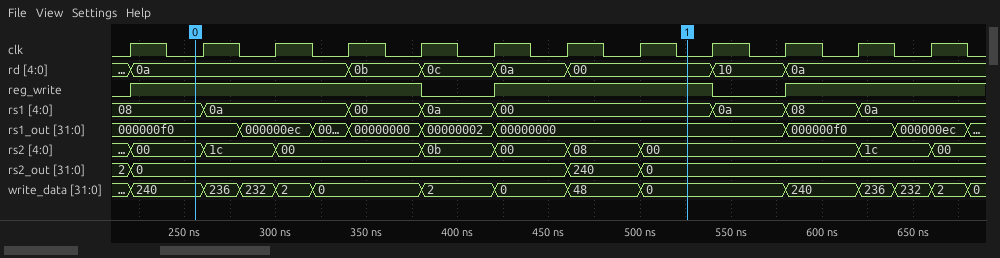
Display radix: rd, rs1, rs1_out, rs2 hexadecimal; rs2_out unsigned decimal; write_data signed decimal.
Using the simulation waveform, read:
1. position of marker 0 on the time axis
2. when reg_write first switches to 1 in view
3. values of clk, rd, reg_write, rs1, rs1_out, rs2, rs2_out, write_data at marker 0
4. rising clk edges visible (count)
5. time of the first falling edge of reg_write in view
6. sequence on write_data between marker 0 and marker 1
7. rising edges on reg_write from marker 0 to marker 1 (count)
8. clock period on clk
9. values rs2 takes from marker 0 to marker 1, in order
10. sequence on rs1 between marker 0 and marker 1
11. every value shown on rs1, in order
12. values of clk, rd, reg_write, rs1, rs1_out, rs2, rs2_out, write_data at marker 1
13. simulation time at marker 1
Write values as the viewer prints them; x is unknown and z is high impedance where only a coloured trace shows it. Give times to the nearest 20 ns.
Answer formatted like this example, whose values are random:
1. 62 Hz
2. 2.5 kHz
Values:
1. 260 ns
2. 220 ns
3. clk=0, rd=0a, reg_write=1, rs1=08, rs1_out=000000f0, rs2=00, rs2_out=0, write_data=240
4. 12
5. 380 ns
6. 240, 236, 232, 2, 0, 2, 0, 48, 0
7. 1
8. 40 ns
9. 00, 1c, 00, 0b, 00, 08, 00
10. 08, 0a, 00, 0a, 00
11. 08, 0a, 00, 0a, 00, 0a, 08, 0a
12. clk=0, rd=00, reg_write=1, rs1=00, rs1_out=00000000, rs2=00, rs2_out=0, write_data=0
13. 520 ns
